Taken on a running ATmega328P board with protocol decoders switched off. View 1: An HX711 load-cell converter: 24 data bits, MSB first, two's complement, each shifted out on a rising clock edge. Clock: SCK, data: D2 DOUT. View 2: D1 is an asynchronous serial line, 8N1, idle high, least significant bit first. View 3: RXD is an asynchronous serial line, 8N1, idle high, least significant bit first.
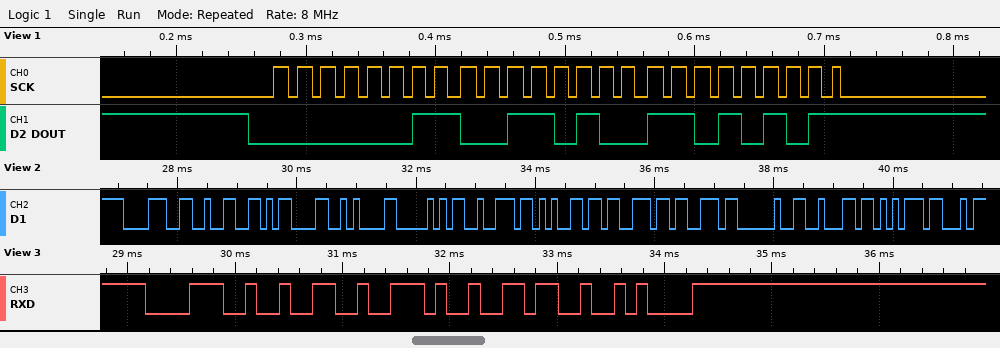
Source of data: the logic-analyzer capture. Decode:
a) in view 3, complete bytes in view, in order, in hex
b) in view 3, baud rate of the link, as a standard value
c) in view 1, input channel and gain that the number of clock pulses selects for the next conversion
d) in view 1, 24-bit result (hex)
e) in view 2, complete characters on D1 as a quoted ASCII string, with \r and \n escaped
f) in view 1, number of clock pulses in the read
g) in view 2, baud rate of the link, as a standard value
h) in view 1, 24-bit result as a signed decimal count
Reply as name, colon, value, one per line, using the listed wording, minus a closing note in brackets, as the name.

in view 3, complete bytes in view, in order, in hex: 0x38 0x32 0x2E 0x36 0x0A
in view 3, baud rate of the link, as a standard value: 9600 baud
in view 1, input channel and gain that the number of clock pulses selects for the next conversion: channel A, gain 128
in view 1, 24-bit result: 0x0334D5
in view 2, complete characters on D1 as a quoted ASCII string, with \r and \n escaped: "82\r\nPress bu"
in view 1, number of clock pulses in the read: 25
in view 2, baud rate of the link, as a standard value: 9600 baud
in view 1, 24-bit result as a signed decimal count: 210133
